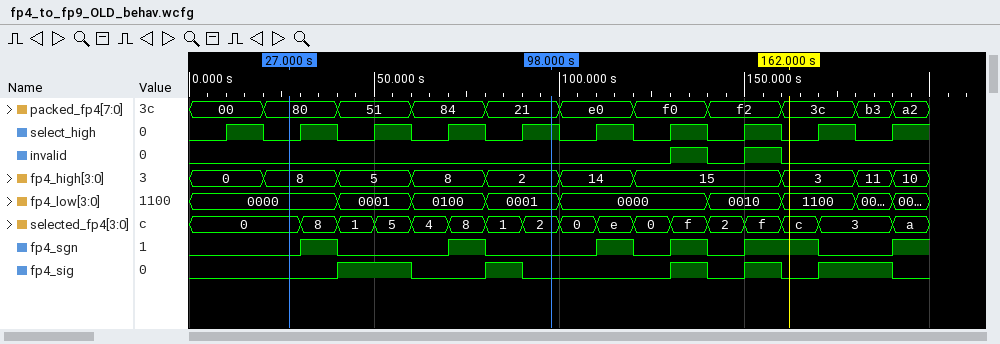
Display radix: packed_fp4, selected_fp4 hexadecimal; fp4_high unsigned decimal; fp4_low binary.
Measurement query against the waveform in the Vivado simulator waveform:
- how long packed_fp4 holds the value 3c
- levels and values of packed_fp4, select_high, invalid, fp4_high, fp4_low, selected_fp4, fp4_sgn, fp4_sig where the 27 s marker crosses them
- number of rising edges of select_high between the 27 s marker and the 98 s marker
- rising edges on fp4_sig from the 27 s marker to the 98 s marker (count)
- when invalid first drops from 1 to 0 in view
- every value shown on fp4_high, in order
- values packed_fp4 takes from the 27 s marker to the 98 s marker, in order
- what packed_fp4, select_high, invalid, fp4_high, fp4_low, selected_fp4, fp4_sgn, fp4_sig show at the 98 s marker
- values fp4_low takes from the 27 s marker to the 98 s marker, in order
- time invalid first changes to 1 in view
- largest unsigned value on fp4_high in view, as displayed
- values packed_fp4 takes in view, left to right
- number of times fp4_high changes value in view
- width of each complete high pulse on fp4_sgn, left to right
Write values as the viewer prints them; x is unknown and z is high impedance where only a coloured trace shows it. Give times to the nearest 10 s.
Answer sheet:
20 s
packed_fp4=80, select_high=0, invalid=0, fp4_high=8, fp4_low=0000, selected_fp4=0, fp4_sgn=0, fp4_sig=0
4
2
140 s
0, 8, 5, 8, 2, 14, 15, 3, 11, 10
80, 51, 84, 21
packed_fp4=21, select_high=1, invalid=0, fp4_high=2, fp4_low=0001, selected_fp4=2, fp4_sgn=0, fp4_sig=0
0000, 0001, 0100, 0001
130 s
15
00, 80, 51, 84, 21, e0, f0, f2, 3c, b3, a2
9
10 s, 10 s, 10 s, 10 s, 20 s
